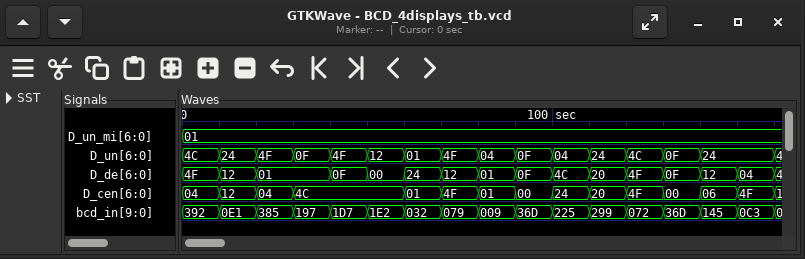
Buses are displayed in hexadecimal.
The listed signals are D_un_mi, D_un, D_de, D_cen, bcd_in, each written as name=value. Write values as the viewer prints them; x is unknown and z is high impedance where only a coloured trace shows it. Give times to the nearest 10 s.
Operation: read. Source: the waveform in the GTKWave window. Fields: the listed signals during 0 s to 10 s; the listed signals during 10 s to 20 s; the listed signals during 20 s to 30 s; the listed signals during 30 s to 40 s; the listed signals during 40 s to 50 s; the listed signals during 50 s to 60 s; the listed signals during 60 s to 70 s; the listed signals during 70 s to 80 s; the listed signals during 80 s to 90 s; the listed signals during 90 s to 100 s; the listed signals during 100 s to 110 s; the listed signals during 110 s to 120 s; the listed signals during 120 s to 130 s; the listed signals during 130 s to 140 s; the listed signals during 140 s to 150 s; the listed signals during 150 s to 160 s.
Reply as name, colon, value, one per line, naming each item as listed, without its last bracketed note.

the listed signals during 0 s to 10 s: D_un_mi=01, D_un=4C, D_de=4F, D_cen=04, bcd_in=392
the listed signals during 10 s to 20 s: D_un_mi=01, D_un=24, D_de=12, D_cen=12, bcd_in=0E1
the listed signals during 20 s to 30 s: D_un_mi=01, D_un=4F, D_de=01, D_cen=04, bcd_in=385
the listed signals during 30 s to 40 s: D_un_mi=01, D_un=0F, D_de=01, D_cen=4C, bcd_in=197
the listed signals during 40 s to 50 s: D_un_mi=01, D_un=4F, D_de=0F, D_cen=4C, bcd_in=1D7
the listed signals during 50 s to 60 s: D_un_mi=01, D_un=12, D_de=00, D_cen=4C, bcd_in=1E2
the listed signals during 60 s to 70 s: D_un_mi=01, D_un=01, D_de=24, D_cen=01, bcd_in=032
the listed signals during 70 s to 80 s: D_un_mi=01, D_un=4F, D_de=12, D_cen=4F, bcd_in=079
the listed signals during 80 s to 90 s: D_un_mi=01, D_un=04, D_de=01, D_cen=01, bcd_in=009
the listed signals during 90 s to 100 s: D_un_mi=01, D_un=0F, D_de=0F, D_cen=00, bcd_in=36D
the listed signals during 100 s to 110 s: D_un_mi=01, D_un=04, D_de=4C, D_cen=24, bcd_in=225
the listed signals during 110 s to 120 s: D_un_mi=01, D_un=24, D_de=20, D_cen=20, bcd_in=299
the listed signals during 120 s to 130 s: D_un_mi=01, D_un=4C, D_de=4F, D_cen=4F, bcd_in=072
the listed signals during 130 s to 140 s: D_un_mi=01, D_un=0F, D_de=0F, D_cen=00, bcd_in=36D
the listed signals during 140 s to 150 s: D_un_mi=01, D_un=24, D_de=12, D_cen=06, bcd_in=145
the listed signals during 150 s to 160 s: D_un_mi=01, D_un=24, D_de=04, D_cen=4F, bcd_in=0C3
